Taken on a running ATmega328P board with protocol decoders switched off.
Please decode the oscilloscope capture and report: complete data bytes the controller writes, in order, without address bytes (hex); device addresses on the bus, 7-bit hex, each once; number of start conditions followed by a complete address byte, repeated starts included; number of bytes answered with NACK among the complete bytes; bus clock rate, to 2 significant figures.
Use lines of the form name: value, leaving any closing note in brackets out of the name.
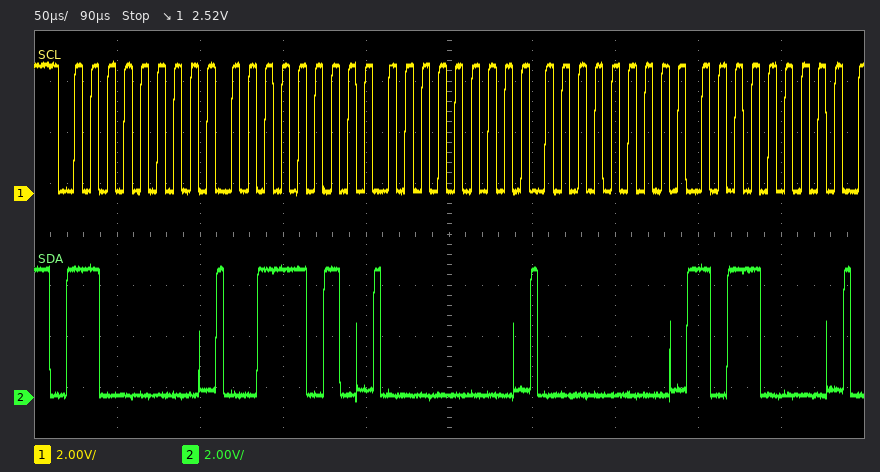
complete data bytes the controller writes, in order, without address bytes: 3A 00 00 B0
device addresses on the bus, 7-bit hex, each once: 0x60
number of start conditions followed by a complete address byte, repeated starts included: 1
number of bytes answered with NACK among the complete bytes: 0
bus clock rate, to 2 significant figures: 100 kHz
